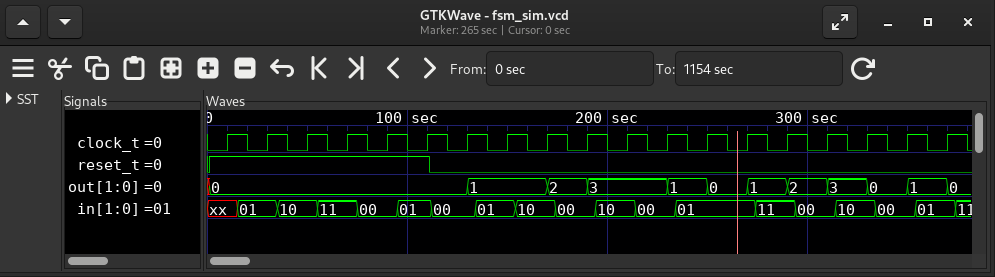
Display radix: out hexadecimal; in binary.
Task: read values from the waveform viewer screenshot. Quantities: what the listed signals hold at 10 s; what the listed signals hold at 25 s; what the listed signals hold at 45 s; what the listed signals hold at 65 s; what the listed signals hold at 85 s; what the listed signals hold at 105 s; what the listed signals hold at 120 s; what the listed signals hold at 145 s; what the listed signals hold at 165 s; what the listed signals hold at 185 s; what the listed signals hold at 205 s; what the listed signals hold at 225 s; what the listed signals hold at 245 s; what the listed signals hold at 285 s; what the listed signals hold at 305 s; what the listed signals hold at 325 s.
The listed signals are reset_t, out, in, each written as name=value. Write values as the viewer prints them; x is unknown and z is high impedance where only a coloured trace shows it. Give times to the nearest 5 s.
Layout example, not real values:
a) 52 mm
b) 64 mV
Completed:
a) reset_t=1, out=0, in=xx
b) reset_t=1, out=0, in=01
c) reset_t=1, out=0, in=10
d) reset_t=1, out=0, in=11
e) reset_t=1, out=0, in=00
f) reset_t=1, out=0, in=01
g) reset_t=0, out=0, in=00
h) reset_t=0, out=1, in=01
i) reset_t=0, out=1, in=10
j) reset_t=0, out=2, in=00
k) reset_t=0, out=3, in=10
l) reset_t=0, out=3, in=00
m) reset_t=0, out=1, in=01
n) reset_t=0, out=1, in=11
o) reset_t=0, out=2, in=00
p) reset_t=0, out=3, in=10
